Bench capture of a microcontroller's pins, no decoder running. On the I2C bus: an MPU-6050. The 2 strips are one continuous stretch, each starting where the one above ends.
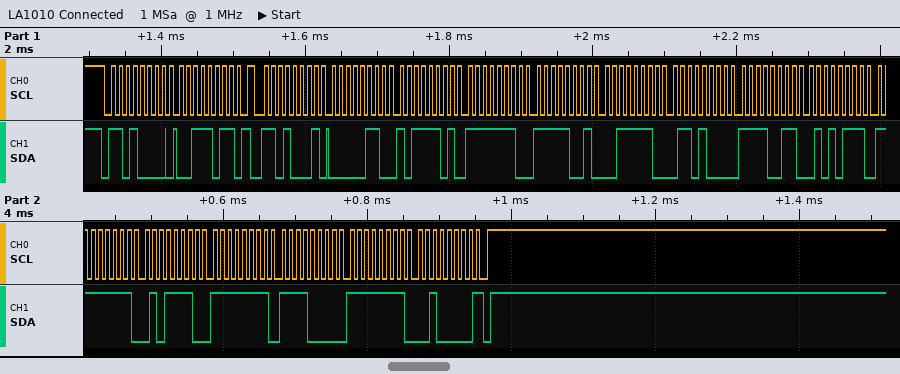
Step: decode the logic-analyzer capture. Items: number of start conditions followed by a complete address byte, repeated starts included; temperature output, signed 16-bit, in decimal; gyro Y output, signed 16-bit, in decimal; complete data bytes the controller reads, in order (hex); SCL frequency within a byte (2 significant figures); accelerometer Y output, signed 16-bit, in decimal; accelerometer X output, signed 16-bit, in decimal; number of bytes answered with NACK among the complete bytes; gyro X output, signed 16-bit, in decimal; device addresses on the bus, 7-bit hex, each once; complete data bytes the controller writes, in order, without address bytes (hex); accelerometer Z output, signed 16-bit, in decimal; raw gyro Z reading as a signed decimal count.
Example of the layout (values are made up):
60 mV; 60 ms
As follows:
2; -3241; -16; 06 BD FE F9 3E 68 F3 57 FF 5E FF F0 FF 20; 100 kHz; -263; 1725; 1; -162; 0x68; 3B; 15976; -224
